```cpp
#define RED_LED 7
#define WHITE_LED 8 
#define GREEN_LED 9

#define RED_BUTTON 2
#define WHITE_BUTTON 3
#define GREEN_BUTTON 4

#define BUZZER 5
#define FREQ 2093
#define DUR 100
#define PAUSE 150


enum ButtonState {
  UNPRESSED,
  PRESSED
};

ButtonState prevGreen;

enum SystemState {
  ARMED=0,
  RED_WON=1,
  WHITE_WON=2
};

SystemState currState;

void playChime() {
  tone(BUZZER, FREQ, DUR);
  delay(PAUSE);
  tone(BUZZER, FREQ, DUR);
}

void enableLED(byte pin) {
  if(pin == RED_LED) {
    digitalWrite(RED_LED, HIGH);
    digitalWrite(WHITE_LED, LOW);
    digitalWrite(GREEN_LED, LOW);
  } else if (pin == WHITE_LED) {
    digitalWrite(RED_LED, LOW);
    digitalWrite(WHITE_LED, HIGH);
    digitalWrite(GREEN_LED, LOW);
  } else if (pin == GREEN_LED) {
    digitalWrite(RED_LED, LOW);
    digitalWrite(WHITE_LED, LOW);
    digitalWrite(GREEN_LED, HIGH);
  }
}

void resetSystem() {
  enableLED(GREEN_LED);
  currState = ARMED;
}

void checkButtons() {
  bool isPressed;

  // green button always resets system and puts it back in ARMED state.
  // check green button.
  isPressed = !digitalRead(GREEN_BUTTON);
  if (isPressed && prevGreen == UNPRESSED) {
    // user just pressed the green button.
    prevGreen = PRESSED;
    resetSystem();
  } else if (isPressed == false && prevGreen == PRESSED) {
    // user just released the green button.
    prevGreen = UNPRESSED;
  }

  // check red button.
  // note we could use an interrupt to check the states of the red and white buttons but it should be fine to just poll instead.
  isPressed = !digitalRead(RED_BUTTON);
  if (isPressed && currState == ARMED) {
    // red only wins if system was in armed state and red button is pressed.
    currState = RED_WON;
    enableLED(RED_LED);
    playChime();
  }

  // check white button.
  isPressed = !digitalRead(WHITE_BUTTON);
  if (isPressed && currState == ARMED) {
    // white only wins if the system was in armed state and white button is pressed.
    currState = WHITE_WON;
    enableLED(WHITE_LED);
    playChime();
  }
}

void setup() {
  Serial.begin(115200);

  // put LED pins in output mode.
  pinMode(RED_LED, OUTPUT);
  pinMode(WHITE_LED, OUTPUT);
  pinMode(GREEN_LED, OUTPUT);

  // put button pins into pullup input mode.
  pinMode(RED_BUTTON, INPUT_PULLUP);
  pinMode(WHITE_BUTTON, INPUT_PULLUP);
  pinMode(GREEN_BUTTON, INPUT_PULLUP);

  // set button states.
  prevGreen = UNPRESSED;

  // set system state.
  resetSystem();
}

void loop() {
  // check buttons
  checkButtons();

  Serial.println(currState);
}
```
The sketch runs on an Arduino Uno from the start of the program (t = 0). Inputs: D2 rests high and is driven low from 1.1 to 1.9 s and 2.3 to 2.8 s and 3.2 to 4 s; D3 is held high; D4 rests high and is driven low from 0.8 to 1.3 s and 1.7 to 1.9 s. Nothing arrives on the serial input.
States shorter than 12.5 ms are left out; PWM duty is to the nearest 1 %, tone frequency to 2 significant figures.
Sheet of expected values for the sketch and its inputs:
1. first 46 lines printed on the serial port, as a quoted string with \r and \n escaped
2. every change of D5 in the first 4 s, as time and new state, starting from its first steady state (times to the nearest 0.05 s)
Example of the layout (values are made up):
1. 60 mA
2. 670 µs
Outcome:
1. "0\r\n0\r\n0\r\n0\r\n0\r\n0\r\n0\r\n0\r\n0\r\n0\r\n0\r\n0\r\n0\r\n0\r\n0\r\n0\r\n0\r\n0\r\n0\r\n0\r\n0\r\n0\r\n0\r\n0\r\n0\r\n0\r\n0\r\n0\r\n0\r\n0\r\n0\r\n0\r\n0\r\n0\r\n0\r\n0\r\n0\r\n0\r\n0\r\n0\r\n0\r\n0\r\n0\r\n0\r\n0\r\n0\r\n"
2. 1.1 s tone 2100 Hz; 1.2 s low; 1.25 s tone 2100 Hz; 1.35 s low; 1.7 s tone 2100 Hz; 1.8 s low; 1.85 s tone 2100 Hz; 1.95 s low
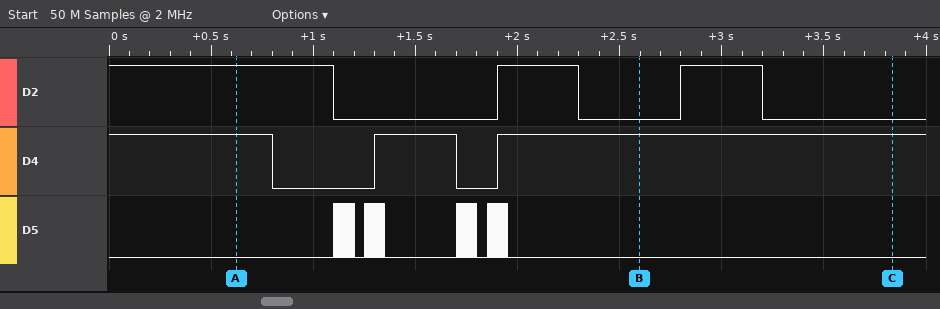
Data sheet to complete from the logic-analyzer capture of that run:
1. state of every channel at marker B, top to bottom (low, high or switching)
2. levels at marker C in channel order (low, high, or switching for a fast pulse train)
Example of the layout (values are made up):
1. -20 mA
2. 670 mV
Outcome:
1. D2 low, D4 high, D5 low
2. D2 low, D4 high, D5 low
